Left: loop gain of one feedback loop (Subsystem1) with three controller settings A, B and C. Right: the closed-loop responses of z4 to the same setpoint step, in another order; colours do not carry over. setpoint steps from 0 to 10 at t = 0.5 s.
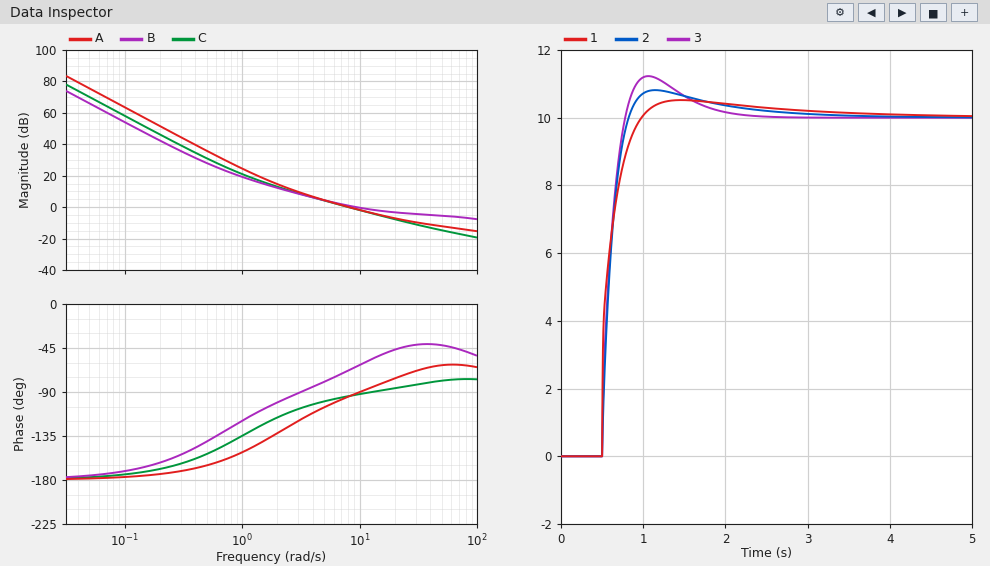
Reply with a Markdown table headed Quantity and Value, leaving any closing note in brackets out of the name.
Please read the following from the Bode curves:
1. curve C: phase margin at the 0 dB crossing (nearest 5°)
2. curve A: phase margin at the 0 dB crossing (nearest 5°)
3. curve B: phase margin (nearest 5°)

| Quantity | Value |
|---|---|
| curve C: phase margin at the 0 dB crossing | 85° |
| curve A: phase margin at the 0 dB crossing | 85° |
| curve B: phase margin | 115° |
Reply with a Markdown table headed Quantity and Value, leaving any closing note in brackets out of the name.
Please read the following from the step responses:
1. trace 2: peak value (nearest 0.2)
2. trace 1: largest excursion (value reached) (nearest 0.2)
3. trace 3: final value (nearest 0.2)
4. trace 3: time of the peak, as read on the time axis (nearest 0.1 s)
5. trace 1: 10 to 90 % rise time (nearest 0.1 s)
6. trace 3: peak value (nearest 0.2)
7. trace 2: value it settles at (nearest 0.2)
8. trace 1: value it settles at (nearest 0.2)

| Quantity | Value |
|---|---|
| trace 2: peak value | 10.8 |
| trace 1: largest excursion (value reached) | 10.6 |
| trace 3: final value | 10.0 |
| trace 3: time of the peak, as read on the time axis | 1.1 s |
| trace 1: 10 to 90 % rise time | 0.3 s |
| trace 3: peak value | 11.2 |
| trace 2: value it settles at | 10.0 |
| trace 1: value it settles at | 10.0 |
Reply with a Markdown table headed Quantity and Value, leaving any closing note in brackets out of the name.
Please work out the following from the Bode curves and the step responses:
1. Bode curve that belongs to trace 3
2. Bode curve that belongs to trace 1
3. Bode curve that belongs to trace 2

| Quantity | Value |
|---|---|
| Bode curve that belongs to trace 3 | A |
| Bode curve that belongs to trace 1 | B |
| Bode curve that belongs to trace 2 | C |
